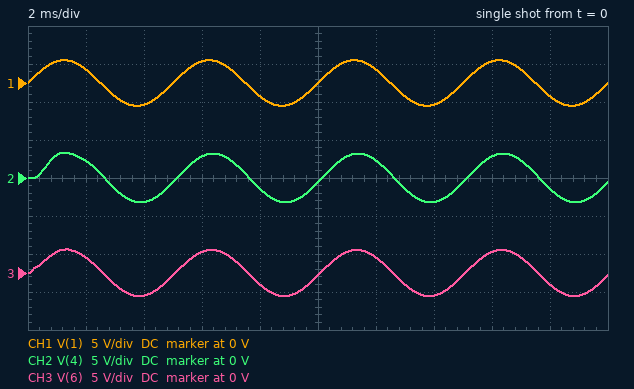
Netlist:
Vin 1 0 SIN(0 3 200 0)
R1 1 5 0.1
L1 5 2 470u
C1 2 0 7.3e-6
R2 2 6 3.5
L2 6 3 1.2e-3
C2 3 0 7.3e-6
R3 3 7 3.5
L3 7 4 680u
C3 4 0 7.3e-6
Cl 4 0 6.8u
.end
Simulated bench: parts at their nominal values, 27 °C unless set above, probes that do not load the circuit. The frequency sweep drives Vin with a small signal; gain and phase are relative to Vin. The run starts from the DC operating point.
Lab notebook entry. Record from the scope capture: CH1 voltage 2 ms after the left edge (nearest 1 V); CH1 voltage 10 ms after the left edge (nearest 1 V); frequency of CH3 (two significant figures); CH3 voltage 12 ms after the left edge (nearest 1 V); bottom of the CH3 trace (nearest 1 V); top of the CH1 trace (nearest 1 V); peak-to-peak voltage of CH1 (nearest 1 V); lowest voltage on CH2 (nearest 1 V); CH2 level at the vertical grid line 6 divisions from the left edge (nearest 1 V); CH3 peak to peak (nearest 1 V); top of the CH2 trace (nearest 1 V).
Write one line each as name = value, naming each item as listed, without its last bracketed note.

CH1 voltage 2 ms after the left edge = 2 V
CH1 voltage 10 ms after the left edge = 0 V
frequency of CH3 = 200 Hz
CH3 voltage 12 ms after the left edge = 2 V
bottom of the CH3 trace = -3 V
top of the CH1 trace = 3 V
peak-to-peak voltage of CH1 = 6 V
lowest voltage on CH2 = -3 V
CH2 level at the vertical grid line 6 divisions from the left edge = 2 V
CH3 peak to peak = 6 V
top of the CH2 trace = 3 V
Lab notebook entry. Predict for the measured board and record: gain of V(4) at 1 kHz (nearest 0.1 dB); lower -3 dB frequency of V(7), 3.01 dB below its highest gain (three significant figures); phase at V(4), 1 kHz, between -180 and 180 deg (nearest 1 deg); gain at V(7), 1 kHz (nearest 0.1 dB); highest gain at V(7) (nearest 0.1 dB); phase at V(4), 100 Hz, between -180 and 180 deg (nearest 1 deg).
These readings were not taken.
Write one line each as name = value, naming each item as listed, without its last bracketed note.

gain of V(4) at 1 kHz = 2.0 dB
lower -3 dB frequency of V(7), 3.01 dB below its highest gain = 2.65 kHz
phase at V(4), 1 kHz, between -180 and 180 deg = -141 deg
gain at V(7), 1 kHz = -2.1 dB
highest gain at V(7) = 7.9 dB
phase at V(4), 100 Hz, between -180 and 180 deg = -5 deg
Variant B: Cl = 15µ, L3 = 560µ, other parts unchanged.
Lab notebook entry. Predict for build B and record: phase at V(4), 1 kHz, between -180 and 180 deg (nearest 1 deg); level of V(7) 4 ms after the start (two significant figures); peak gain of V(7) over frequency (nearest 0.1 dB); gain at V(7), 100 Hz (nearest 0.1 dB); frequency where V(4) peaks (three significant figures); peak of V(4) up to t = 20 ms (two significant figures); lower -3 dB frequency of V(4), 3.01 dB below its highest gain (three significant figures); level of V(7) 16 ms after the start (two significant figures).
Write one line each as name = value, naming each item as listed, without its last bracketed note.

phase at V(4), 1 kHz, between -180 and 180 deg = -149 deg
level of V(7) 4 ms after the start = -3.2 V
peak gain of V(7) over frequency = 6.9 dB
gain at V(7), 100 Hz = 0.1 dB
frequency where V(4) peaks = 584 Hz
peak of V(4) up to t = 20 ms = 3.4 V
lower -3 dB frequency of V(4), 3.01 dB below its highest gain = 279 Hz
level of V(7) 16 ms after the start = 2.7 V
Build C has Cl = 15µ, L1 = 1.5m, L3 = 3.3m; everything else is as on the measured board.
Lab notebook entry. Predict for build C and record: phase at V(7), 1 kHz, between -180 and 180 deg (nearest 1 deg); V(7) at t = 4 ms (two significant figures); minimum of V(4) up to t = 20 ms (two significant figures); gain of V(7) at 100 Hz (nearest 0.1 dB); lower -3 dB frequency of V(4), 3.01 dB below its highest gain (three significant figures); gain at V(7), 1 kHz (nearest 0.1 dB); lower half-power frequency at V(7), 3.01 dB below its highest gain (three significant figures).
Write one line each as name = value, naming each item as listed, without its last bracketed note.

phase at V(7), 1 kHz, between -180 and 180 deg = 2 deg
V(7) at t = 4 ms = -3.5 V
minimum of V(4) up to t = 20 ms = -3.9 V
gain of V(7) at 100 Hz = 0.3 dB
lower -3 dB frequency of V(4), 3.01 dB below its highest gain = 299 Hz
gain at V(7), 1 kHz = 0.2 dB
lower half-power frequency at V(7), 3.01 dB below its highest gain = 1.28 kHz
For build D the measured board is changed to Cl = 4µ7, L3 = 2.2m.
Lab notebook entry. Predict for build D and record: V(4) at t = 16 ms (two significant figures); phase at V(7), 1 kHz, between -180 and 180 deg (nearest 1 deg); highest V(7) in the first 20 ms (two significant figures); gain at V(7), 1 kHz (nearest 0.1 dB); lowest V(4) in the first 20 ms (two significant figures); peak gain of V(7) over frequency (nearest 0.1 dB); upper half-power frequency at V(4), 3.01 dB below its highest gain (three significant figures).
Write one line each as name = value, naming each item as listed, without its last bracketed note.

V(4) at t = 16 ms = 2.9 V
phase at V(7), 1 kHz, between -180 and 180 deg = 24 deg
highest V(7) in the first 20 ms = 3.4 V
gain at V(7), 1 kHz = -26.0 dB
lowest V(4) in the first 20 ms = -3.3 V
peak gain of V(7) over frequency = 14.4 dB
upper half-power frequency at V(4), 3.01 dB below its highest gain = 820 Hz
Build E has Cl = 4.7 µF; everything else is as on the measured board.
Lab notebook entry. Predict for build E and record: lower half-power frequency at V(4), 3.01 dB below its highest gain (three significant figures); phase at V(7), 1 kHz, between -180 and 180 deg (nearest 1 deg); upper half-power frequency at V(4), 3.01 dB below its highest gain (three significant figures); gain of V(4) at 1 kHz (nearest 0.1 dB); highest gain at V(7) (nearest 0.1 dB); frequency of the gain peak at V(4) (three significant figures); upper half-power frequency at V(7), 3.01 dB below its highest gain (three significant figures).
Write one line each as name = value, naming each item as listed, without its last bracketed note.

lower half-power frequency at V(4), 3.01 dB below its highest gain = 549 Hz
phase at V(7), 1 kHz, between -180 and 180 deg = -136 deg
upper half-power frequency at V(4), 3.01 dB below its highest gain = 974 Hz
gain of V(4) at 1 kHz = 3.8 dB
highest gain at V(7) = 7.4 dB
frequency of the gain peak at V(4) = 776 Hz
upper half-power frequency at V(7), 3.01 dB below its highest gain = 3.67 kHz
